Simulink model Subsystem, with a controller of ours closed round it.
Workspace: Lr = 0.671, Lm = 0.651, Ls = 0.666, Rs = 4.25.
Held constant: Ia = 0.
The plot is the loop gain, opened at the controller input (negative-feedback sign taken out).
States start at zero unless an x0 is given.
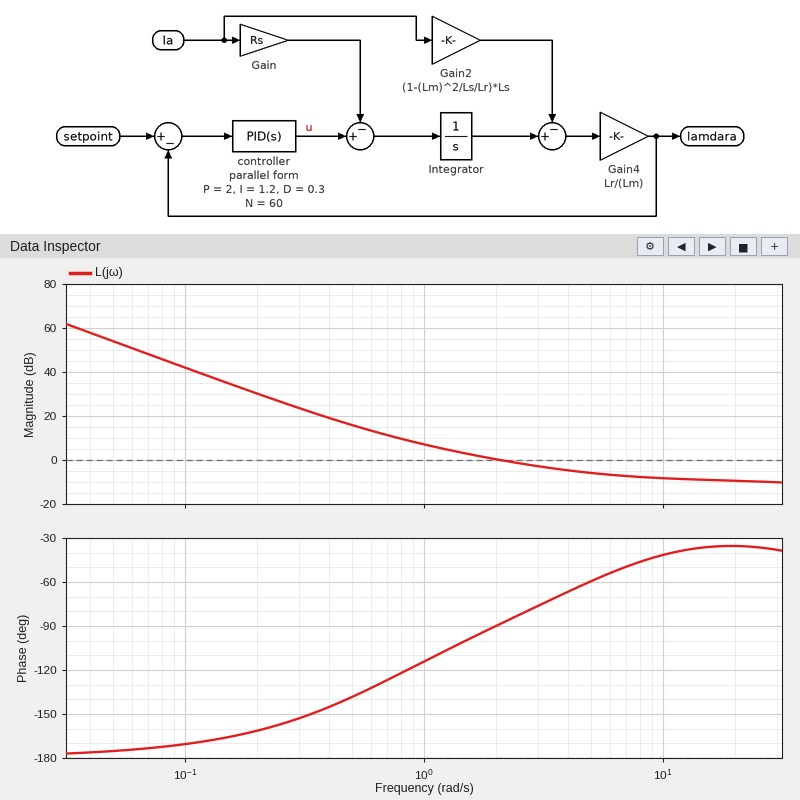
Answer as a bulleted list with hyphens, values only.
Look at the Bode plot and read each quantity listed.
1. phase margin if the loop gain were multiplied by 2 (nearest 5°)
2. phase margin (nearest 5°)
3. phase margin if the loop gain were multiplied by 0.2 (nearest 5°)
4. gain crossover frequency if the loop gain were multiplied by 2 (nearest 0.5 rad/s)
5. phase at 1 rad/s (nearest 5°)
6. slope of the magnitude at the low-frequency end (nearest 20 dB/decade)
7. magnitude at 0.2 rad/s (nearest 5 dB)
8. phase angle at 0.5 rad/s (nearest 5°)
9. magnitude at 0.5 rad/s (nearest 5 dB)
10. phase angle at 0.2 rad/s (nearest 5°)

- 120°
- 90°
- 45°
- 5.0 rad/s
- -115°
- -40 dB/decade
- 30 dB
- -140°
- 15 dB
- -160°
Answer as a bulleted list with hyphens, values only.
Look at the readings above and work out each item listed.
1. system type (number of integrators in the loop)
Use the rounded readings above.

- 2
